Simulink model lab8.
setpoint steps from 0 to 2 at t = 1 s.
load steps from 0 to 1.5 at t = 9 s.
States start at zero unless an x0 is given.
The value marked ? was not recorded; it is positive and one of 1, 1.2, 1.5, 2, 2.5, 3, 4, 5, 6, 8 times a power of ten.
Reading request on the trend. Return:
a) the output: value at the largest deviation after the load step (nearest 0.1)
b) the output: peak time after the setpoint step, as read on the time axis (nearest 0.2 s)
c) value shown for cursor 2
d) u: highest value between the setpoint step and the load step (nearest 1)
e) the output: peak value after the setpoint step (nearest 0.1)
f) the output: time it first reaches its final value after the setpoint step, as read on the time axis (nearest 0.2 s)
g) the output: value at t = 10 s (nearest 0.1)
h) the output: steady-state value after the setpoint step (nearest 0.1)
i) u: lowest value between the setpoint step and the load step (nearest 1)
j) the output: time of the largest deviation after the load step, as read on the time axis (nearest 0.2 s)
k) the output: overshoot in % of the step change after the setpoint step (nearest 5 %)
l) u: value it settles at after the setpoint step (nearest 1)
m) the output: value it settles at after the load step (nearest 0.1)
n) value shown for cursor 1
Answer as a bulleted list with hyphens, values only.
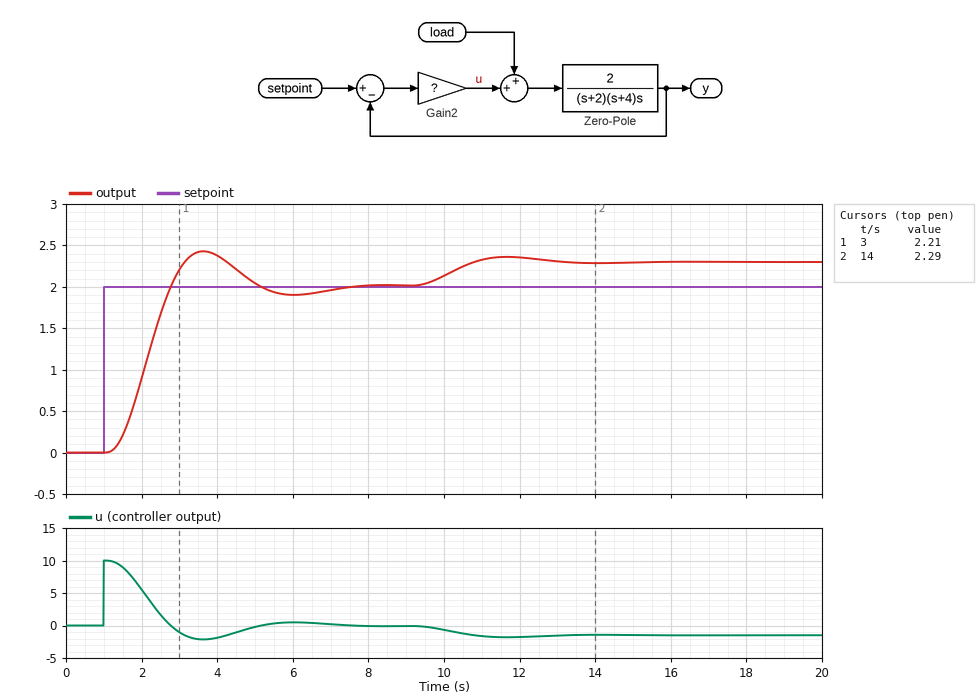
- 2.4
- 3.6 s
- 2.29
- 10
- 2.4
- 2.8 s
- 2.1
- 2.0
- -2
- 11.6 s
- 20 %
- 0
- 2.3
- 2.21
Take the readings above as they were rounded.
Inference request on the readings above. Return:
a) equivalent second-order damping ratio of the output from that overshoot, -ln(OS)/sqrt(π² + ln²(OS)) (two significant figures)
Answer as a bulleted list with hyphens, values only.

- 0.46
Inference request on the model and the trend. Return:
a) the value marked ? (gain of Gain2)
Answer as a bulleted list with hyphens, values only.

- 5
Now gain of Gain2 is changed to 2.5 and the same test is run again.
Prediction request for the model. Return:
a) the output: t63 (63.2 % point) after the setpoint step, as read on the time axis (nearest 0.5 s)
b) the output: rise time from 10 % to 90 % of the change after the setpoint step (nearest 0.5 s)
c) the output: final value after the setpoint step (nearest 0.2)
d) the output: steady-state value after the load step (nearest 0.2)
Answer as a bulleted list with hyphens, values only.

- 3.0 s
- 2.0 s
- 2.0
- 2.6
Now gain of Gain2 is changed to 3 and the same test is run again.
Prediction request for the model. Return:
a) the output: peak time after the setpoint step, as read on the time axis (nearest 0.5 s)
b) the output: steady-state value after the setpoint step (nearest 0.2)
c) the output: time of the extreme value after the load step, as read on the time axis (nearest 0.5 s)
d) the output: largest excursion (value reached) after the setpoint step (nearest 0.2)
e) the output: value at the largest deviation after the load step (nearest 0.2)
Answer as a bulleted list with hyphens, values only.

- 5.0 s
- 2.0
- 13.0 s
- 2.2
- 2.6
